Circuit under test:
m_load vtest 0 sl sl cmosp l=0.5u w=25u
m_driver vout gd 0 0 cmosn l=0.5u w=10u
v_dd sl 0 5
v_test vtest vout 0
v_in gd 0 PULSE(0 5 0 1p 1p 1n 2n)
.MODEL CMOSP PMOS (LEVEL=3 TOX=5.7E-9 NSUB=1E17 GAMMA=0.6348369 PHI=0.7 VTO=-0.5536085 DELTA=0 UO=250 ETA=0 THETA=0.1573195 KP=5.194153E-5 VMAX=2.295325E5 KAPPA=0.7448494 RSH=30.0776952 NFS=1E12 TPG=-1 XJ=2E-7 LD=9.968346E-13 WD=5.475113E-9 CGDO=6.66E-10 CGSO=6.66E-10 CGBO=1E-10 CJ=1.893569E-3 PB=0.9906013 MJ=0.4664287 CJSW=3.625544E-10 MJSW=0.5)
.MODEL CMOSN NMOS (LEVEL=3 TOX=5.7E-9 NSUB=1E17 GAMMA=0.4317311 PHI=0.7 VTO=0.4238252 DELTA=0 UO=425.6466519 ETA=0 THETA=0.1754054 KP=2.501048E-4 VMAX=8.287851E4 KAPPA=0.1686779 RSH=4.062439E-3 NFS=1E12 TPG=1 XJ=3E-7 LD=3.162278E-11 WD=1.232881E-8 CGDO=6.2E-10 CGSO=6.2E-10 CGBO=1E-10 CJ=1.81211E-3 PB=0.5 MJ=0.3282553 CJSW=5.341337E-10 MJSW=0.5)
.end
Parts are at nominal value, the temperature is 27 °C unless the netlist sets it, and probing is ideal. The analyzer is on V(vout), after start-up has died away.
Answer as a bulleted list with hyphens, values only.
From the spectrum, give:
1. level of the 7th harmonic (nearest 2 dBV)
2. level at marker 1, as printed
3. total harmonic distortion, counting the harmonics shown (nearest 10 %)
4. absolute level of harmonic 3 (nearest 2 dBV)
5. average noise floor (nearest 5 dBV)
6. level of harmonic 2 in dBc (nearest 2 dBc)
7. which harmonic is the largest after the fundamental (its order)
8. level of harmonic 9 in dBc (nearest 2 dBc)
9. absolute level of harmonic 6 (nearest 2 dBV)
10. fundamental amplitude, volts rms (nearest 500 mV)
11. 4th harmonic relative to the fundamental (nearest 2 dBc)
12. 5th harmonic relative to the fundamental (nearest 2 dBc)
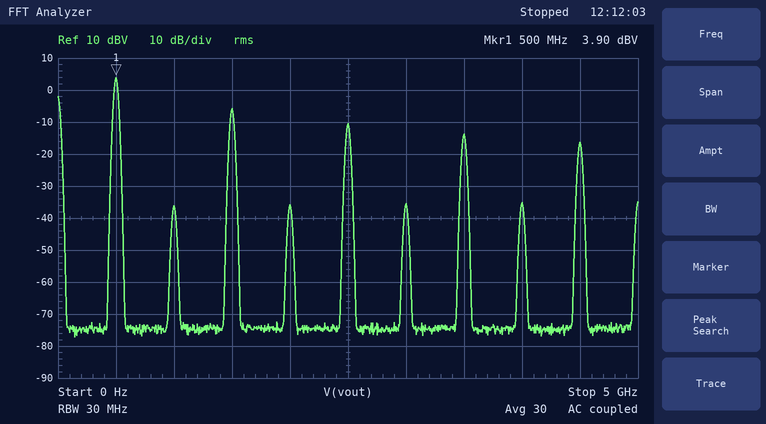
- -14 dBV
- 3.90 dBV
- 40 %
- -6 dBV
- -75 dBV
- -40 dBc
- 3
- -20 dBc
- -36 dBV
- 1.5 V
- -40 dBc
- -14 dBc
